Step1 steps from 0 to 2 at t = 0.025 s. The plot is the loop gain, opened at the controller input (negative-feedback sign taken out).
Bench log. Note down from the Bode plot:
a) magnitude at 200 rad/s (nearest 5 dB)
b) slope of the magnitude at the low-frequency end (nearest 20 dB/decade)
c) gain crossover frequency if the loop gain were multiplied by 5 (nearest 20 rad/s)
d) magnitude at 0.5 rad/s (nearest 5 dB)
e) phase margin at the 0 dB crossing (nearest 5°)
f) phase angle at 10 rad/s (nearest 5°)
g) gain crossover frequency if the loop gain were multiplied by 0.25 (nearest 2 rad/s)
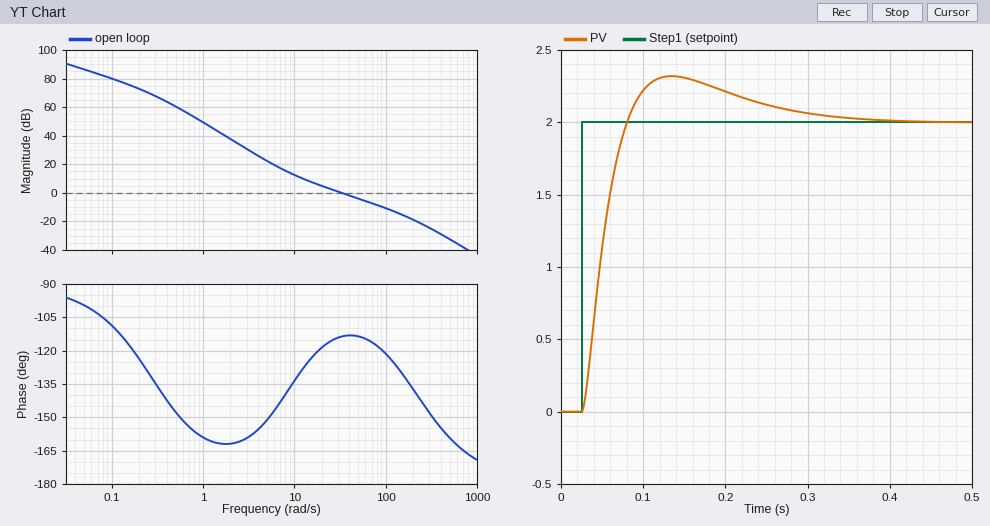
-20 dB
-20 dB/decade
140 rad/s
60 dB
65°
-135°
10 rad/s
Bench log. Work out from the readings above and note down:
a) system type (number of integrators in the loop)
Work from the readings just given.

1
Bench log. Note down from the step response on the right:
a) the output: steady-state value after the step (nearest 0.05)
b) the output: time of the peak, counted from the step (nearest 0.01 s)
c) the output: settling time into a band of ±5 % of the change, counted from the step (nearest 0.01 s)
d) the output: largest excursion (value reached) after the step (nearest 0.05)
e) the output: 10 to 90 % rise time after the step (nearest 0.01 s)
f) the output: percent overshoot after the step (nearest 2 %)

2.00
0.11 s
0.24 s
2.30
0.04 s
16 %
